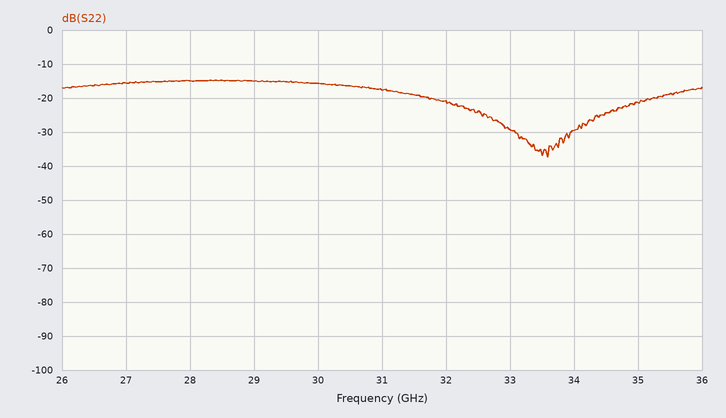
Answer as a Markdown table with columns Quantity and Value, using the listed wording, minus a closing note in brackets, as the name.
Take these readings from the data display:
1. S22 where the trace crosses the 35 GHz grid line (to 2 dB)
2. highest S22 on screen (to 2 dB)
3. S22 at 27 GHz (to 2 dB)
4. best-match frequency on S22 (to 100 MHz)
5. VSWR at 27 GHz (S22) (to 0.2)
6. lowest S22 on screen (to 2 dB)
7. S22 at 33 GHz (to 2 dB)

| Quantity | Value |
|---|---|
| S22 where the trace crosses the 35 GHz grid line | -22 dB |
| highest S22 on screen | -14 dB |
| S22 at 27 GHz | -16 dB |
| best-match frequency on S22 | 33.6 GHz |
| VSWR at 27 GHz (S22) | 1.4 |
| lowest S22 on screen | -38 dB |
| S22 at 33 GHz | -30 dB |
